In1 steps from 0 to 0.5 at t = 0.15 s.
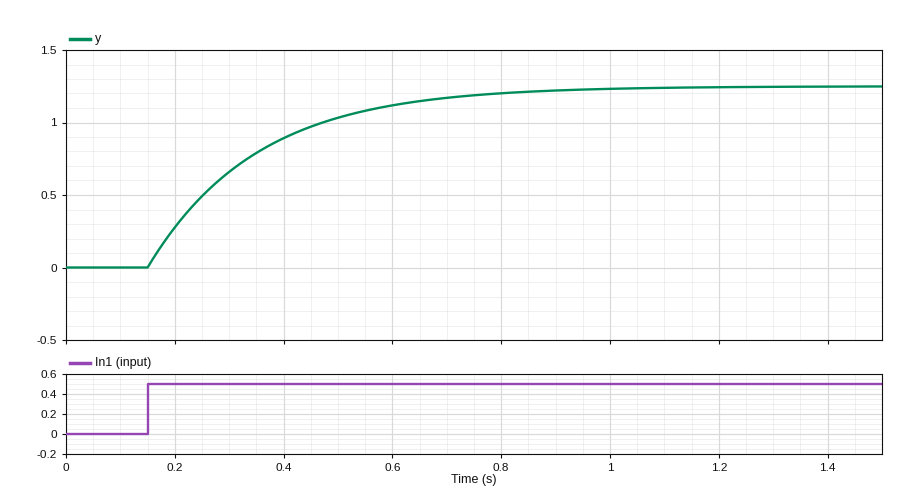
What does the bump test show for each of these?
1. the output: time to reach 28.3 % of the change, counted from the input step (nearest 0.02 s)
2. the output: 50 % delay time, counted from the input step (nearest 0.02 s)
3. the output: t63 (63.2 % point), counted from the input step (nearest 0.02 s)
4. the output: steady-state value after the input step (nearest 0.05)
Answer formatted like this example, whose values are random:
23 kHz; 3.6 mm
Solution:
0.06 s; 0.14 s; 0.20 s; 1.25
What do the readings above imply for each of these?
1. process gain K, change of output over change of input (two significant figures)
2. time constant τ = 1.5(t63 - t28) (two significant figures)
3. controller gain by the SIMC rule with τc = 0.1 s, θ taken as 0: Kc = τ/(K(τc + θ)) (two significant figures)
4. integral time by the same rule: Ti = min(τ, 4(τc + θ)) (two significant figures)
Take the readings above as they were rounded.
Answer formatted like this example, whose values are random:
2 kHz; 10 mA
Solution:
2.5; 0.21 s; 0.84; 0.21 s
